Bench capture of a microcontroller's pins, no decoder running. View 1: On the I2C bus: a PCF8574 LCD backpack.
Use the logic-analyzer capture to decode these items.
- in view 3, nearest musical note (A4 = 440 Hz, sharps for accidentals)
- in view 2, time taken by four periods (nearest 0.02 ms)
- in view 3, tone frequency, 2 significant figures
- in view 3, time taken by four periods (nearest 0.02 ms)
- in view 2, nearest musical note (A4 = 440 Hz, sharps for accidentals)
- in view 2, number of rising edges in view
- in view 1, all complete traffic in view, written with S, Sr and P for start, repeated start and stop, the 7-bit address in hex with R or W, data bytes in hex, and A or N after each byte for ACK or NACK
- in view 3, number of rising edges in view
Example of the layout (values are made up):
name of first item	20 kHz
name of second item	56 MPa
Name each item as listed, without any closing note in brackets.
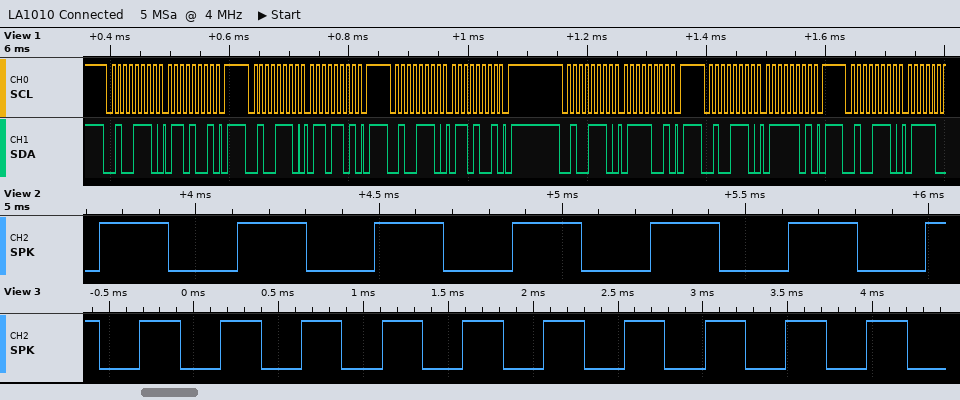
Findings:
in view 3, nearest musical note	C7
in view 2, time taken by four periods	1.50 ms
in view 3, tone frequency, 2 significant figures	2.1 kHz
in view 3, time taken by four periods	1.90 ms
in view 2, nearest musical note	E7
in view 2, number of rising edges in view	7
in view 1, all complete traffic in view, written with S, Sr and P for start, repeated start and stop, the 7-bit address in hex with R or W, data bytes in hex, and A or N after each byte for ACK or NACK	S 27W A 69 A P S 27W A 6D A P S 27W A 69 A P S 27W A 79 A P S 27W A 7D A P S 27W A
in view 3, number of rising edges in view	10
